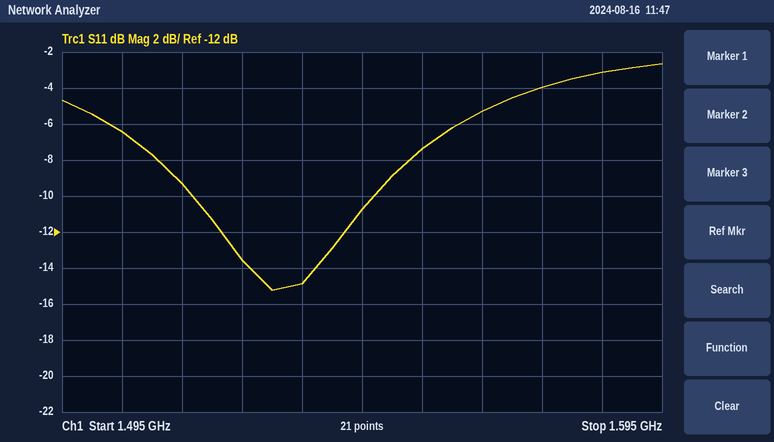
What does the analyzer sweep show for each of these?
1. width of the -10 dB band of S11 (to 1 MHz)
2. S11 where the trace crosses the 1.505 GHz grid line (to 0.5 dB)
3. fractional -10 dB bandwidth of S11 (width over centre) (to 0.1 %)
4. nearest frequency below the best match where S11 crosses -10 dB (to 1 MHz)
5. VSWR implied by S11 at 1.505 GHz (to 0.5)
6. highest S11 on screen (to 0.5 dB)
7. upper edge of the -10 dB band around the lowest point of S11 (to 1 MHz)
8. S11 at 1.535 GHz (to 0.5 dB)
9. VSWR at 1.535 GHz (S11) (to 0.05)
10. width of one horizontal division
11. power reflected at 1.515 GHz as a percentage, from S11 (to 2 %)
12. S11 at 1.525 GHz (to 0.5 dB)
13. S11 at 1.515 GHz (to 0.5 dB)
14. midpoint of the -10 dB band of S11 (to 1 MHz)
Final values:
30 MHz
-6.5 dB
2.0 %
1.517 GHz
3.0
-2.5 dB
1.547 GHz
-15.0 dB
1.45
10 MHz
12 %
-13.5 dB
-9.5 dB
1.532 GHz
